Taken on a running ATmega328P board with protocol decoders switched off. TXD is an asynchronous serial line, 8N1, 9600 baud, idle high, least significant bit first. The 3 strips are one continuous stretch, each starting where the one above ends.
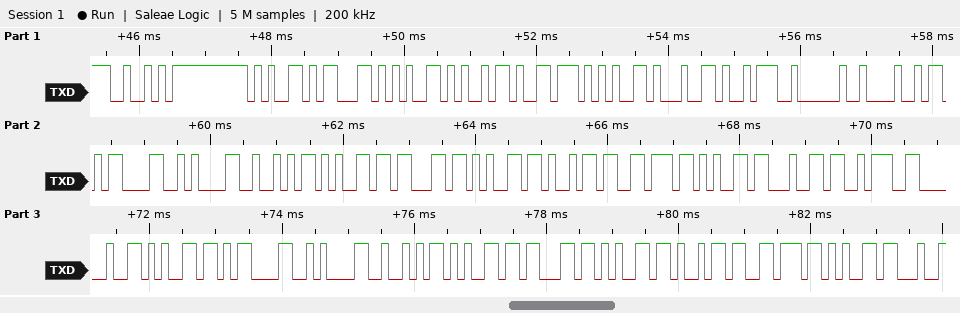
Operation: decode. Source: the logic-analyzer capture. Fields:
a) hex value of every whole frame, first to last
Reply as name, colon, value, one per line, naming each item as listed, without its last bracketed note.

hex value of every whole frame, first to last: 52 65 63 65 69 76 65 64 3A 20 48 0D 0A 52 65 63 65 69 76 65 64 3A 20 65 0D 0A 52 65 63 65 69 76 65
